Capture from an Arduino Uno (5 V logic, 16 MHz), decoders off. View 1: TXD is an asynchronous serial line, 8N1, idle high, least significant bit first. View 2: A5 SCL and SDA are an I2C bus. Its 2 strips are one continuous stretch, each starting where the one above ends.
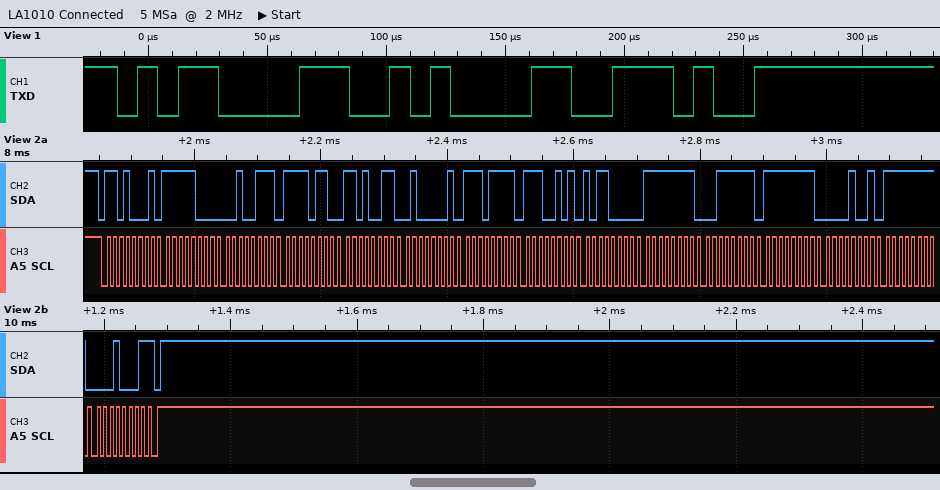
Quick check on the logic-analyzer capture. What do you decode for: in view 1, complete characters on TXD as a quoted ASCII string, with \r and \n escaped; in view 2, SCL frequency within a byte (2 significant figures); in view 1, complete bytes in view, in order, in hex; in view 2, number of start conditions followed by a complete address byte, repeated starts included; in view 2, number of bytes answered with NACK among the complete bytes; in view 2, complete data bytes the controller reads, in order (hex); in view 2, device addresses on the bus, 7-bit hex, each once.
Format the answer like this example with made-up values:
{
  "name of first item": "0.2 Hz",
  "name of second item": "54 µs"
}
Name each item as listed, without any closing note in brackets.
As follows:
{
  "in view 1, complete characters on TXD as a quoted ASCII string, with \\r and \\n escaped": "\"\\r\\n.\"",
  "in view 2, SCL frequency within a byte": "100 kHz",
  "in view 1, complete bytes in view, in order, in hex": "0x0D 0x0A 0x2E",
  "in view 2, number of start conditions followed by a complete address byte, repeated starts included": "1",
  "in view 2, number of bytes answered with NACK among the complete bytes": "1",
  "in view 2, complete data bytes the controller reads, in order": "F8 27 F6 D3 41 EF E5 B0 FF 3F FF 09 FF 11",
  "in view 2, device addresses on the bus, 7-bit hex, each once": "0x68"
}
